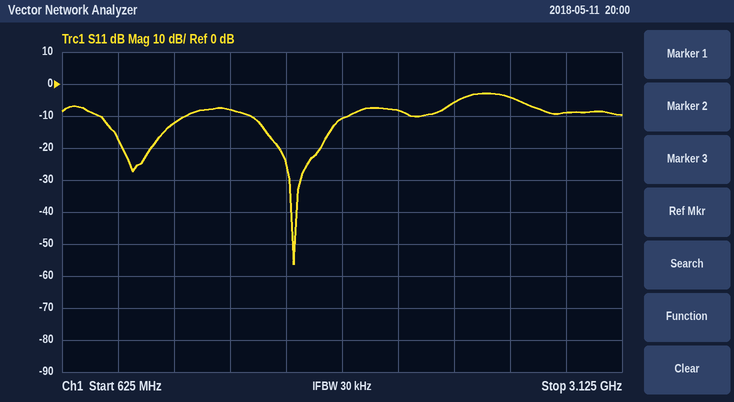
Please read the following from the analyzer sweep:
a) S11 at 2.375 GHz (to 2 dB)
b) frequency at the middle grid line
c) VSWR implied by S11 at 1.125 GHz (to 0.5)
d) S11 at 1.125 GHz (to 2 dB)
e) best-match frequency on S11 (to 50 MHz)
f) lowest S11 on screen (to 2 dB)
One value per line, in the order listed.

-6 dB
1.875 GHz
1.5
-12 dB
1.65 GHz
-56 dB
